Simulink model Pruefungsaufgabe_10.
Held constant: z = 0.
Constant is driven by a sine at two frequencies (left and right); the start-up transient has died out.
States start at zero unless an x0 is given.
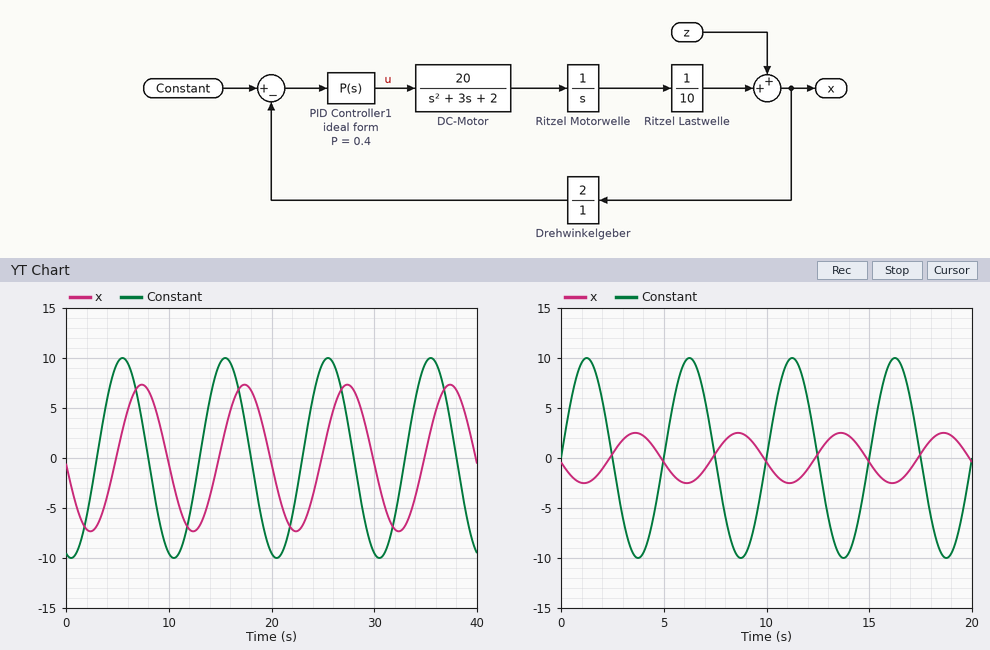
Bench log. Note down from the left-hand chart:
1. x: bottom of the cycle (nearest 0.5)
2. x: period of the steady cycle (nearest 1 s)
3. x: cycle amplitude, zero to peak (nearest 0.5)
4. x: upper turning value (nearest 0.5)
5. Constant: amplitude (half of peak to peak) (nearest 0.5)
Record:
-7.5
10 s
7.5
7.5
10.0
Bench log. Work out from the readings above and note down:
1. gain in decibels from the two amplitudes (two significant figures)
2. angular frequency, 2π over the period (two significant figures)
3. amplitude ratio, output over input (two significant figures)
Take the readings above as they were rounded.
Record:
-2.5 dB
0.63 rad/s
0.75
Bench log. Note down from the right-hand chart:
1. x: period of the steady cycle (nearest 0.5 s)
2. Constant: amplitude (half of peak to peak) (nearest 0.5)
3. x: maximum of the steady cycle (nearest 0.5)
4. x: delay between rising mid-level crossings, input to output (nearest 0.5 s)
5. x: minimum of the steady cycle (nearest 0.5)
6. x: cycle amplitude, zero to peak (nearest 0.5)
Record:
5.0 s
10.0
2.5
2.5 s
-2.5
2.5
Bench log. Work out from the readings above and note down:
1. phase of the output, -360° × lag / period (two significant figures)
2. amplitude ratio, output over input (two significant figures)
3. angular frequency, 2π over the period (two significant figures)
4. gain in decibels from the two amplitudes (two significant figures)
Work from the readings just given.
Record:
-180°
0.25
1.3 rad/s
-12 dB
